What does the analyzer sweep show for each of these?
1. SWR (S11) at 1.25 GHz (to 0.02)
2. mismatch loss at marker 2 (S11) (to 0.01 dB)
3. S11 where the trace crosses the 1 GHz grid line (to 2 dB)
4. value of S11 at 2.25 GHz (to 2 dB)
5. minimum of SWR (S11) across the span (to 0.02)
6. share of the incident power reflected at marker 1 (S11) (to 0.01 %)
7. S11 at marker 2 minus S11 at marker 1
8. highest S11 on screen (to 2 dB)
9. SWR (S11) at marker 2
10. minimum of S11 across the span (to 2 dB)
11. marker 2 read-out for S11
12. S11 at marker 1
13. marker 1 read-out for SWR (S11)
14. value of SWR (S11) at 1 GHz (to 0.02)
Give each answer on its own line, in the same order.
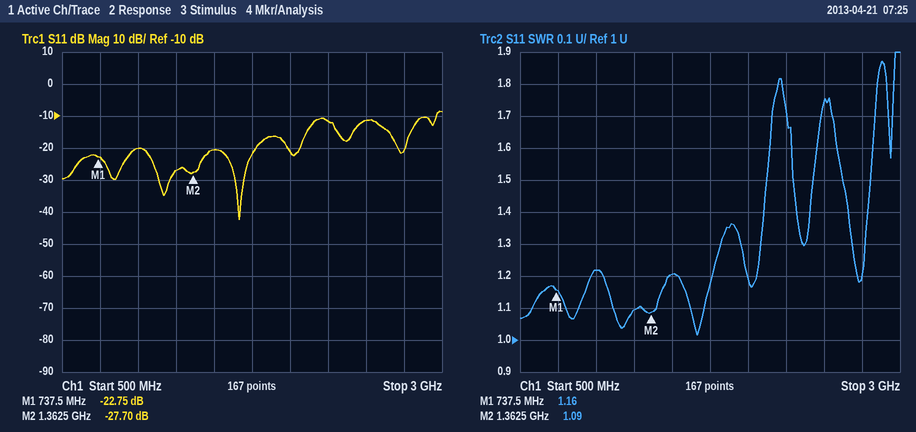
1.10
0.01 dB
-20 dB
-12 dB
1.02
0.53 %
-4.95 dB
-8 dB
1.09
-42 dB
-27.70 dB
-22.75 dB
1.16
1.22
